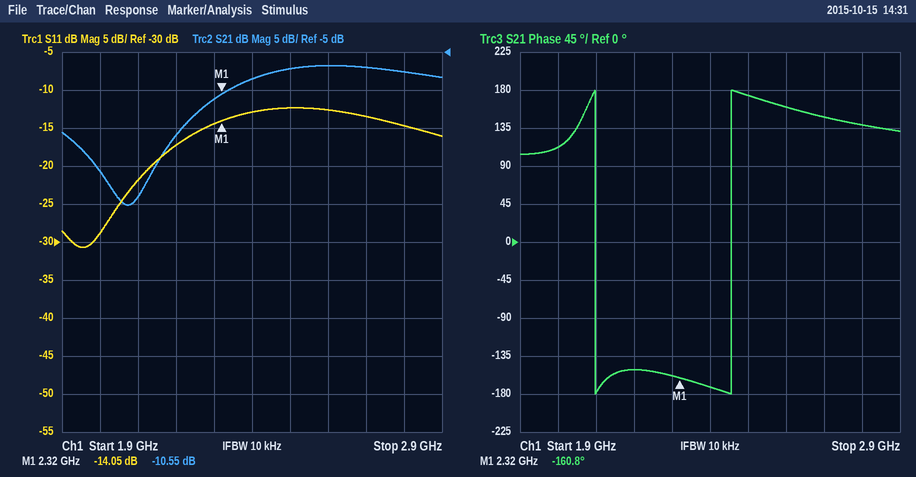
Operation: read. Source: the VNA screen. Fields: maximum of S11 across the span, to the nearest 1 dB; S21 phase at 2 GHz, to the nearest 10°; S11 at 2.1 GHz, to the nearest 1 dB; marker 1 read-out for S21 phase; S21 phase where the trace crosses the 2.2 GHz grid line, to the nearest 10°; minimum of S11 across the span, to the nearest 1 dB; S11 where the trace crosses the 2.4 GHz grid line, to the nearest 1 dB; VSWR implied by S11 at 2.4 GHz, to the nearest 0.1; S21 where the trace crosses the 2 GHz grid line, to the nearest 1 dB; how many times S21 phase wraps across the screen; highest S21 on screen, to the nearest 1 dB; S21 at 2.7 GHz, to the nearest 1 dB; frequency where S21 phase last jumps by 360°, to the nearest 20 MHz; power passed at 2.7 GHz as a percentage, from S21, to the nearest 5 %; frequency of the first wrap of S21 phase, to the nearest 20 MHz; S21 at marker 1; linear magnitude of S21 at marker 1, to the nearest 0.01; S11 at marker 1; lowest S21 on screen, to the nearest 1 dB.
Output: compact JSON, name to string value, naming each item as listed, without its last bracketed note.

{"maximum of S11 across the span, to the nearest 1 dB": "-12 dB", "S21 phase at 2 GHz, to the nearest 10°": "110°", "S11 at 2.1 GHz, to the nearest 1 dB": "-22 dB", "marker 1 read-out for S21 phase": "-160.8°", "S21 phase where the trace crosses the 2.2 GHz grid line, to the nearest 10°": "-150°", "minimum of S11 across the span, to the nearest 1 dB": "-31 dB", "S11 where the trace crosses the 2.4 GHz grid line, to the nearest 1 dB": "-13 dB", "VSWR implied by S11 at 2.4 GHz, to the nearest 0.1": "1.6", "S21 where the trace crosses the 2 GHz grid line, to the nearest 1 dB": "-21 dB", "how many times S21 phase wraps across the screen": "2", "highest S21 on screen, to the nearest 1 dB": "-7 dB", "S21 at 2.7 GHz, to the nearest 1 dB": "-7 dB", "frequency where S21 phase last jumps by 360°, to the nearest 20 MHz": "2.46 GHz", "power passed at 2.7 GHz as a percentage, from S21, to the nearest 5 %": "20 %", "frequency of the first wrap of S21 phase, to the nearest 20 MHz": "2.10 GHz", "S21 at marker 1": "-10.55 dB", "linear magnitude of S21 at marker 1, to the nearest 0.01": "0.30", "S11 at marker 1": "-14.05 dB", "lowest S21 on screen, to the nearest 1 dB": "-25 dB"}
